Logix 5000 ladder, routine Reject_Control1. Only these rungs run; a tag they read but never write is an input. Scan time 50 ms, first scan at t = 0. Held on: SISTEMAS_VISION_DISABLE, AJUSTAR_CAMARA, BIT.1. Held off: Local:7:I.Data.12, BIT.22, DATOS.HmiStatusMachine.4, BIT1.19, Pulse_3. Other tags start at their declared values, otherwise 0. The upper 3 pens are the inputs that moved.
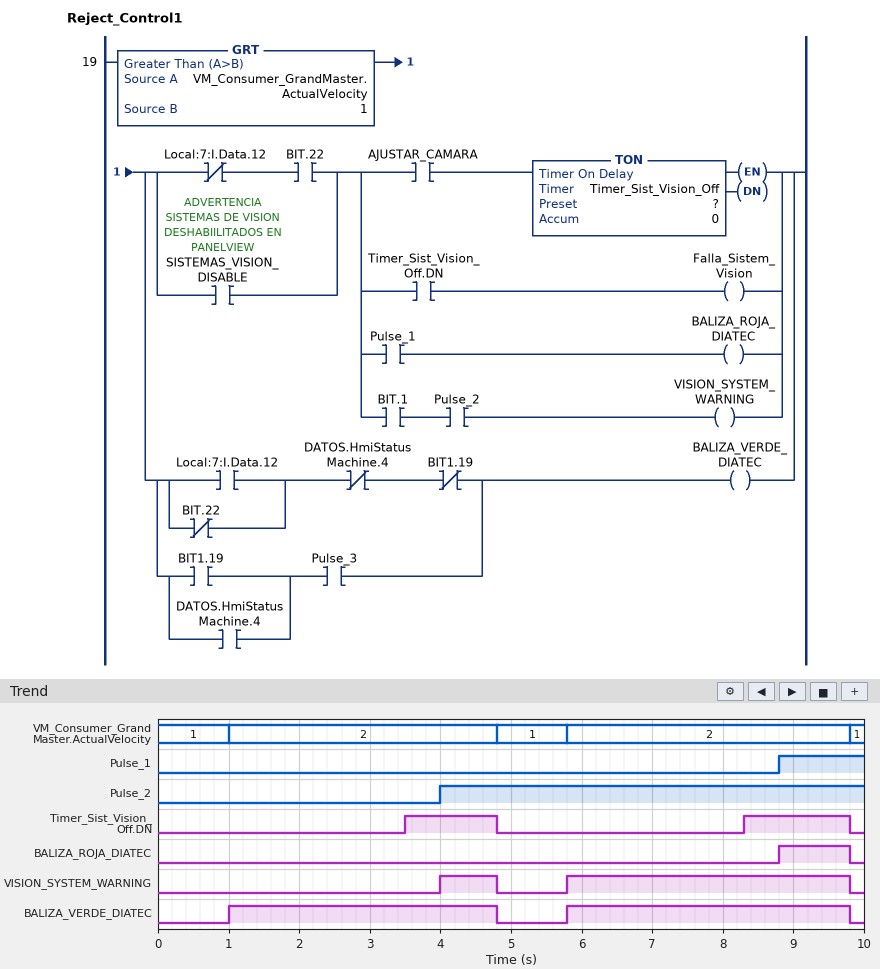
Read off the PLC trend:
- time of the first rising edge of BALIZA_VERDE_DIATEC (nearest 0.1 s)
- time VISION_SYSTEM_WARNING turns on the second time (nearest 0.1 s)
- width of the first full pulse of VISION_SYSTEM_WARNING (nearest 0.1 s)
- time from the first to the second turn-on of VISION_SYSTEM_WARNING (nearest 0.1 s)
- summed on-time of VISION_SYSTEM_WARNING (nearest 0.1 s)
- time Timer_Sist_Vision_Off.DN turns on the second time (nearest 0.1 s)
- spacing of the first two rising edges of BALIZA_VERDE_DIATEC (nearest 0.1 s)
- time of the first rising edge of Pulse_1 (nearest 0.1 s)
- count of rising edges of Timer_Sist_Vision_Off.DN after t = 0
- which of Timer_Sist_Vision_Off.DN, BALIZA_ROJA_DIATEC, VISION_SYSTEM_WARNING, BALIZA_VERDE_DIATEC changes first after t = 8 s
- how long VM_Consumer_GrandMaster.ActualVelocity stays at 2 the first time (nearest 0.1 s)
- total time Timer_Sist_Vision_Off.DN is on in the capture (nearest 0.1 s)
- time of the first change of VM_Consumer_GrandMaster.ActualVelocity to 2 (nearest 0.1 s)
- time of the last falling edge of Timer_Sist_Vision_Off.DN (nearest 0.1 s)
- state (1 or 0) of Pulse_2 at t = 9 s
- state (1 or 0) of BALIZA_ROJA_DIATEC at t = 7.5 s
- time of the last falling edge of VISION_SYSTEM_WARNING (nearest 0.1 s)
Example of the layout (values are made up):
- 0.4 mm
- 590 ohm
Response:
- 1.0 s
- 5.8 s
- 0.8 s
- 1.8 s
- 4.8 s
- 8.3 s
- 4.8 s
- 8.8 s
- 2
- Timer_Sist_Vision_Off.DN
- 3.8 s
- 2.8 s
- 1.0 s
- 9.8 s
- 1
- 0
- 9.8 s
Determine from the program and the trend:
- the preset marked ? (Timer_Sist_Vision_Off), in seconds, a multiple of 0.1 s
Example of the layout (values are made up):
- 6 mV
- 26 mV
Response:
- 2.5 s
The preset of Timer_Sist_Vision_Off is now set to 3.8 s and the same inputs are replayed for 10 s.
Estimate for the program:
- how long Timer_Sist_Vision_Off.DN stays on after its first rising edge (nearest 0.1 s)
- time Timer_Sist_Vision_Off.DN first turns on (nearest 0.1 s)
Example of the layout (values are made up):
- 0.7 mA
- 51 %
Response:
- 0.2 s
- 9.6 s
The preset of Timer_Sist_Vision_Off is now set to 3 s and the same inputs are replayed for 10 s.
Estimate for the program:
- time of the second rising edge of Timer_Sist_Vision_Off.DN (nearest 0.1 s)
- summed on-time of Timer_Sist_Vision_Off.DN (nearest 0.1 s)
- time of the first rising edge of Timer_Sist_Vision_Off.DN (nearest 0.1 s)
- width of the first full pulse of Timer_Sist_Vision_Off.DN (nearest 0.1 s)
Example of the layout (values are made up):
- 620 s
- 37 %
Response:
- 8.8 s
- 1.8 s
- 4.0 s
- 0.8 s
